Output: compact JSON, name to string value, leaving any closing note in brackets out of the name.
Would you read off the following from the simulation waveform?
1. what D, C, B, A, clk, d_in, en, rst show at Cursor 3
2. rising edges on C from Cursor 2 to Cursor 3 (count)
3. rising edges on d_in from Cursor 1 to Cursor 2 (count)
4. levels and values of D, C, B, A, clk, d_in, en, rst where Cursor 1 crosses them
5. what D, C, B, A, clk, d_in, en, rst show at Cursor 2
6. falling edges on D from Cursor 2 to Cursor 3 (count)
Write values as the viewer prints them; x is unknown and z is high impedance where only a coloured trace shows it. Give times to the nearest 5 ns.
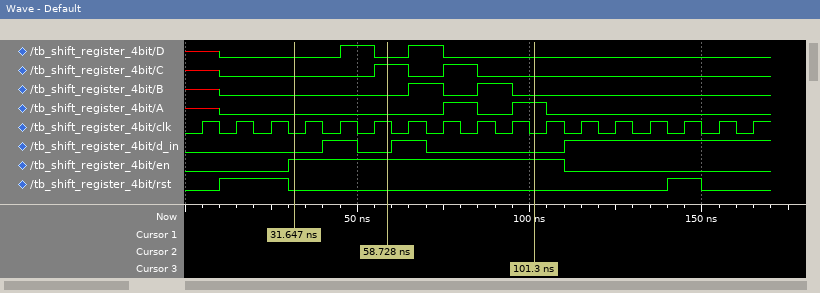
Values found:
{"what D, C, B, A, clk, d_in, en, rst show at Cursor 3": "D=0, C=0, B=0, A=1, clk=0, d_in=0, en=1, rst=0", "rising edges on C from Cursor 2 to Cursor 3": "1", "rising edges on d_in from Cursor 1 to Cursor 2": "1", "levels and values of D, C, B, A, clk, d_in, en, rst where Cursor 1 crosses them": "D=0, C=0, B=0, A=0, clk=0, d_in=0, en=1, rst=0", "what D, C, B, A, clk, d_in, en, rst show at Cursor 2": "D=0, C=1, B=0, A=0, clk=1, d_in=0, en=1, rst=0", "falling edges on D from Cursor 2 to Cursor 3": "1"}
